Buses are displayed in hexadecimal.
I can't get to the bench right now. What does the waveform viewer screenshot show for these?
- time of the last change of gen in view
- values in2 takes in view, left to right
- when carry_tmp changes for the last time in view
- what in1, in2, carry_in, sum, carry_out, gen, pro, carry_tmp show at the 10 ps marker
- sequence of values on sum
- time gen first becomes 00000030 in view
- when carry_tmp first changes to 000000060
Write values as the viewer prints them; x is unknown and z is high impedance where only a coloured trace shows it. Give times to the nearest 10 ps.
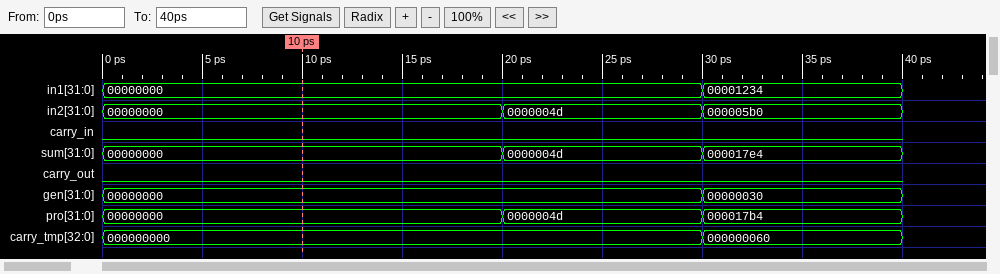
30 ps
00000000, 0000004d, 000005b0
30 ps
in1=00000000, in2=00000000, carry_in=0, sum=00000000, carry_out=0, gen=00000000, pro=00000000, carry_tmp=000000000
00000000, 0000004d, 000017e4
30 ps
30 ps
